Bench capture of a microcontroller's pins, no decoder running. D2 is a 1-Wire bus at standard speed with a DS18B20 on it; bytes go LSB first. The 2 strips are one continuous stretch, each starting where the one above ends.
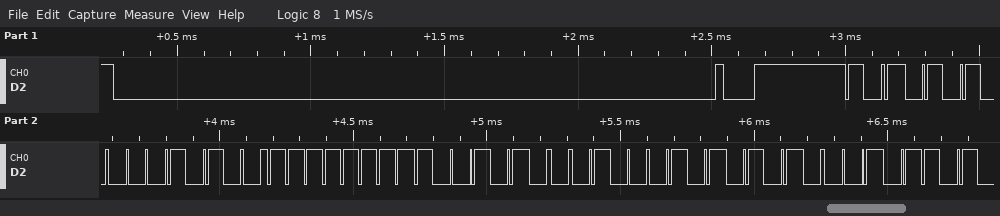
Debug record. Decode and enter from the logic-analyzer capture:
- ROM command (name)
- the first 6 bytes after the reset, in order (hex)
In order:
Match ROM
55 28 FF 29 A2 8A
